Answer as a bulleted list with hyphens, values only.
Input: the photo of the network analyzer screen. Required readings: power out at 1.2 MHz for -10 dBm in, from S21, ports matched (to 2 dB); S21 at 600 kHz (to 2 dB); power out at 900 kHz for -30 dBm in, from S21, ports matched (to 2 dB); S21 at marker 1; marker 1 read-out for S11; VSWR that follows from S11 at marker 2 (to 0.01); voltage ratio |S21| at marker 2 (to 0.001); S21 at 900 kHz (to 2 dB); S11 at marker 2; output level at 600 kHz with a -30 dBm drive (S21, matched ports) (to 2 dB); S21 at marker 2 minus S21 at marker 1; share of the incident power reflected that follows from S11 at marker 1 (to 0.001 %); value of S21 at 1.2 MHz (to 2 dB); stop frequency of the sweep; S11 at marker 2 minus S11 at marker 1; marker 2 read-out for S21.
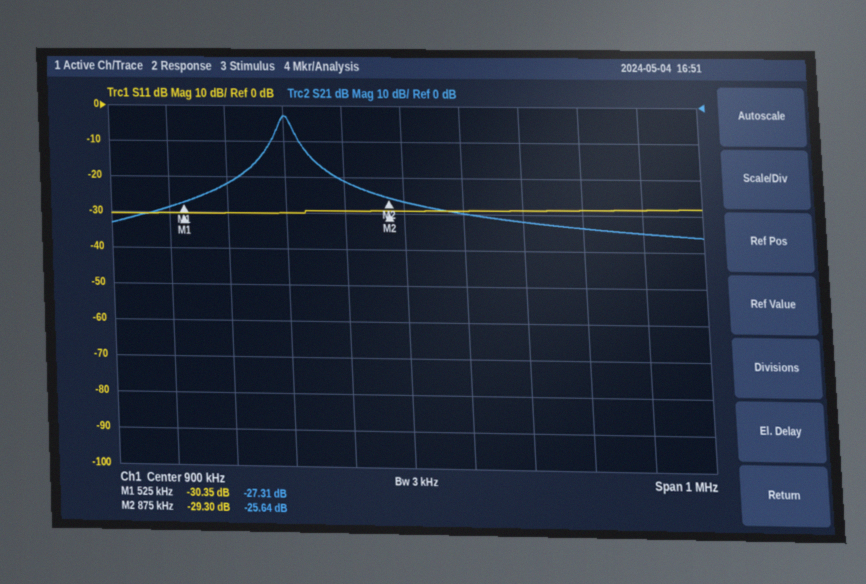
- -44 dBm
- -22 dB
- -56 dBm
- -27.31 dB
- -30.35 dB
- 1.07
- 0.052
- -26 dB
- -29.30 dB
- -52 dBm
- 1.67 dB
- 0.092 %
- -34 dB
- 1.4 MHz
- 1.05 dB
- -25.64 dB
